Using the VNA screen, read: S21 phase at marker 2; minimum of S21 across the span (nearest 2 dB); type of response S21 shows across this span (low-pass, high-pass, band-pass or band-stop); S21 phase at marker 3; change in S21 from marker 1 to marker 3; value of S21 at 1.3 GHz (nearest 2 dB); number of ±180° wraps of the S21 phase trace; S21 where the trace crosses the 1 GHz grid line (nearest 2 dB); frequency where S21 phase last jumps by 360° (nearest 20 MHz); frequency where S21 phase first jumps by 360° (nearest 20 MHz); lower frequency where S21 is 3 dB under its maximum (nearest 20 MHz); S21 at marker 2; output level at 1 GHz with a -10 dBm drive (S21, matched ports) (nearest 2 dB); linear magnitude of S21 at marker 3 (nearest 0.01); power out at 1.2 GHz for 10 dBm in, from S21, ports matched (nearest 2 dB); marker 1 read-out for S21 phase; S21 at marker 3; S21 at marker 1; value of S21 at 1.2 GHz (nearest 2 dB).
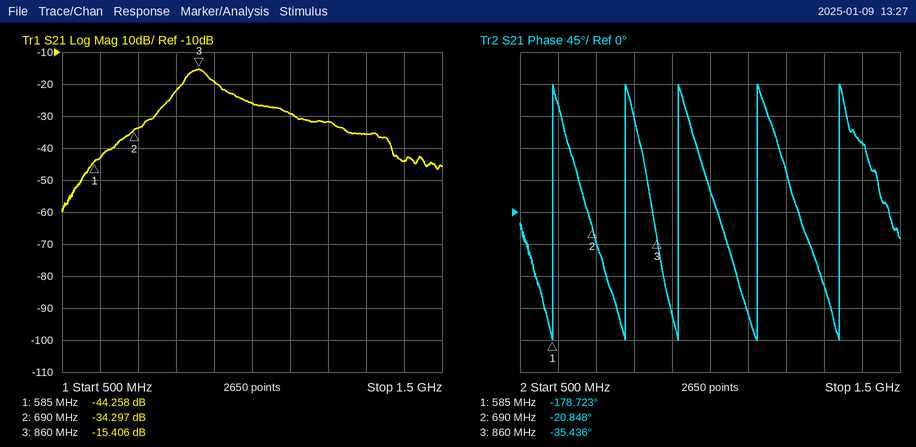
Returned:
-20.848°
-60 dB
band-pass
-35.436°
28.852 dB
-36 dB
5
-26 dB
1.34 GHz
580 MHz
820 MHz
-34.297 dB
-36 dBm
0.17
-22 dBm
-178.723°
-15.406 dB
-44.258 dB
-32 dB
